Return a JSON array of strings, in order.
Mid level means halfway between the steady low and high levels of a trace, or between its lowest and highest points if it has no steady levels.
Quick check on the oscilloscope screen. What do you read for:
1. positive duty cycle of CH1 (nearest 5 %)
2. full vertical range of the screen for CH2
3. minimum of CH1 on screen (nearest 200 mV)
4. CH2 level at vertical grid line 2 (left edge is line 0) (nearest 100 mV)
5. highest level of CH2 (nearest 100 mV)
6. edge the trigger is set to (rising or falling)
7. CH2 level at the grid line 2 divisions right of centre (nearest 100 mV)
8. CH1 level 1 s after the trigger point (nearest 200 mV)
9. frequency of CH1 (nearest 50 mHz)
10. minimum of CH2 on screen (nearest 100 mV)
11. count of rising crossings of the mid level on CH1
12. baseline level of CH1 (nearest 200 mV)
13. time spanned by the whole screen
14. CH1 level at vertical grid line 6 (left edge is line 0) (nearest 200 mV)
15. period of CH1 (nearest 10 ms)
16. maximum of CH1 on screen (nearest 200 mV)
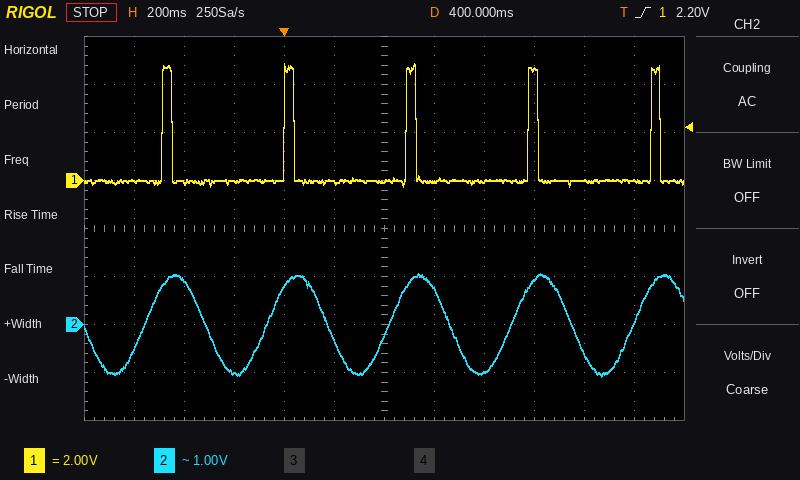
["10 %", "8 V", "-200 mV", "900 mV", "1.1 V", "rising", "-1.0 V", "4.6 V", "2.05 Hz", "-1.1 V", "5", "0.0 V", "2.4 s", "0.0 V", "490 ms", "4.8 V"]
